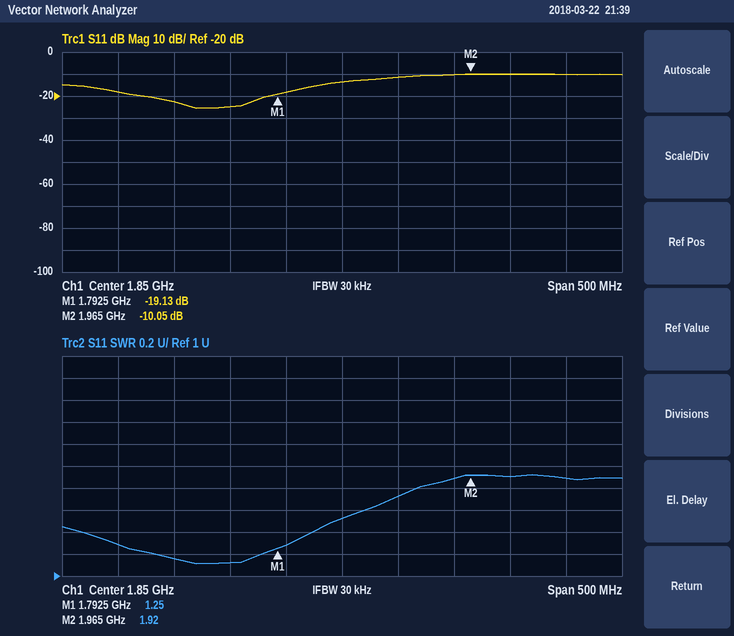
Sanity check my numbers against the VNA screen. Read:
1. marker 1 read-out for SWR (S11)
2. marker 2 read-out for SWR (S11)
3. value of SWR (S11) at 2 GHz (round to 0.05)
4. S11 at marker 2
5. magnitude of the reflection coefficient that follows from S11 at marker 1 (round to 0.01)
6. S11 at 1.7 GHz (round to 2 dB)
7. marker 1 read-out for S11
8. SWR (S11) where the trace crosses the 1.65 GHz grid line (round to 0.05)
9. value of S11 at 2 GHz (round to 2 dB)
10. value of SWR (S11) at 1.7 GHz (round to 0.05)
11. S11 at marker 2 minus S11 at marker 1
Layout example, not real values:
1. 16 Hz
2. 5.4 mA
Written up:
1. 1.25
2. 1.92
3. 1.90
4. -10.05 dB
5. 0.11
6. -22 dB
7. -19.13 dB
8. 1.30
9. -10 dB
10. 1.15
11. 9.08 dB
